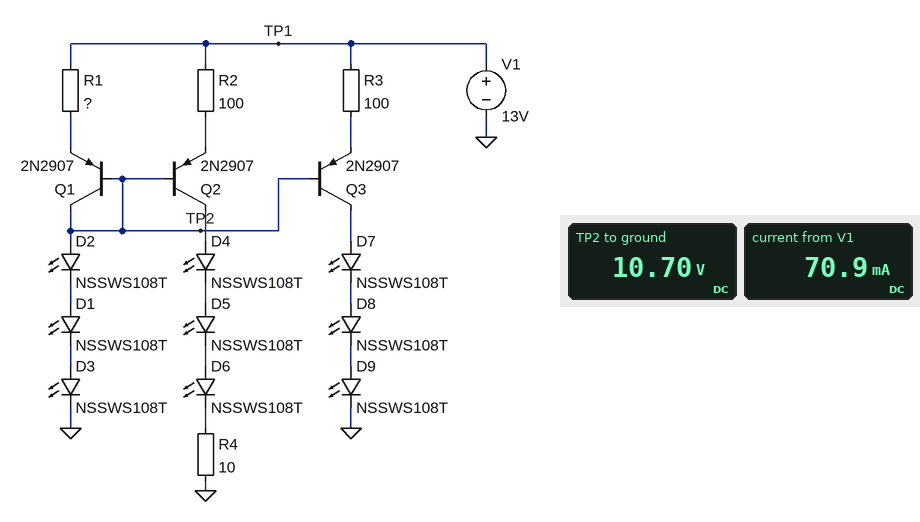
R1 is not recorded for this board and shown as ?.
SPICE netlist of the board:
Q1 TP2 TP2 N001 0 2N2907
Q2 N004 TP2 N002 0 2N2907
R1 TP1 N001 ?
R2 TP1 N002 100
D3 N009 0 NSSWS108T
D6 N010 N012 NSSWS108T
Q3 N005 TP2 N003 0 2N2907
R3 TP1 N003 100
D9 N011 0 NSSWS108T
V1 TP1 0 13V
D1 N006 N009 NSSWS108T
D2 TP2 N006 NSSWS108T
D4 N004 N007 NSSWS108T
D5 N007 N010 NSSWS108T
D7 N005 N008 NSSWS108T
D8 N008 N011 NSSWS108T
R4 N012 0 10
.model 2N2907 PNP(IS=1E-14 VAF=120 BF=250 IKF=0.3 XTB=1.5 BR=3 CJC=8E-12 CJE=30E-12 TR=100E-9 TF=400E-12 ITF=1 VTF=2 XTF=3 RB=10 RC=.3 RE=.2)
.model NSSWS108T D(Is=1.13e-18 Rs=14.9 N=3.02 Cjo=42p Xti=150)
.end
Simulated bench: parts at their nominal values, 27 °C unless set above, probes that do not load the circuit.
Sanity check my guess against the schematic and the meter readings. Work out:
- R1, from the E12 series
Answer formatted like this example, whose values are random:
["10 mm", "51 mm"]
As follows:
["39 Ω"]
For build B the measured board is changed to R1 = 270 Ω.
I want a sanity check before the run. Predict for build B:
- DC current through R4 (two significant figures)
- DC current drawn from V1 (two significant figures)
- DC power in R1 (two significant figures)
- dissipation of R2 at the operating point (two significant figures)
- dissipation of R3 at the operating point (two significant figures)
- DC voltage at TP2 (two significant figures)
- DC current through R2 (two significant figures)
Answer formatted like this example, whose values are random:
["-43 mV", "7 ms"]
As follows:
["24 mA", "67 mA", "31 mW", "79 mW", "81 mW", "9.4 V", "28 mA"]
